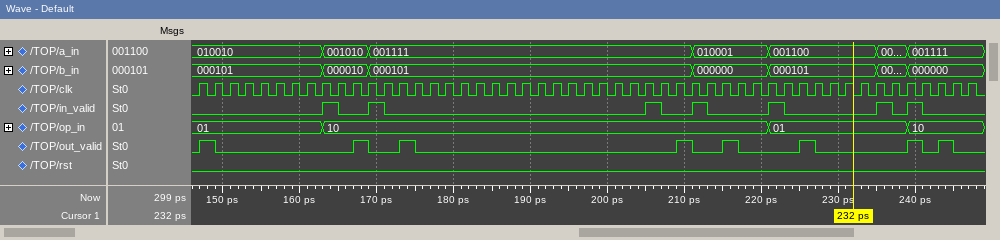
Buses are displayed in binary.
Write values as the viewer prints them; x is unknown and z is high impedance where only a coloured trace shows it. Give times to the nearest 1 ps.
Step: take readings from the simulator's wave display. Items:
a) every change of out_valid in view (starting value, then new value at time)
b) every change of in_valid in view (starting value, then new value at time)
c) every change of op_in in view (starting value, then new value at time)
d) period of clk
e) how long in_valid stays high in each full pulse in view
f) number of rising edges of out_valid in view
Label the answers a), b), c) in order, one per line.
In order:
a) 0, 1 at 147 ps, 0 at 149 ps, 1 at 167 ps, 0 at 169 ps, 1 at 173 ps, 0 at 175 ps, 1 at 209 ps, 0 at 211 ps, 1 at 215 ps, 0 at 217 ps, 1 at 225 ps, 0 at 227 ps, 1 at 239 ps, 0 at 241 ps, 1 at 243 ps, 0 at 245 ps
b) 0, 1 at 163 ps, 0 at 165 ps, 1 at 169 ps, 0 at 171 ps, 1 at 205 ps, 0 at 207 ps, 1 at 211 ps, 0 at 213 ps, 1 at 221 ps, 0 at 223 ps, 1 at 235 ps, 0 at 237 ps, 1 at 239 ps, 0 at 241 ps
c) 01, 10 at 163 ps, 01 at 221 ps, 10 at 239 ps
d) 2 ps
e) 2 ps, 2 ps, 2 ps, 2 ps, 2 ps, 2 ps, 2 ps
f) 8
